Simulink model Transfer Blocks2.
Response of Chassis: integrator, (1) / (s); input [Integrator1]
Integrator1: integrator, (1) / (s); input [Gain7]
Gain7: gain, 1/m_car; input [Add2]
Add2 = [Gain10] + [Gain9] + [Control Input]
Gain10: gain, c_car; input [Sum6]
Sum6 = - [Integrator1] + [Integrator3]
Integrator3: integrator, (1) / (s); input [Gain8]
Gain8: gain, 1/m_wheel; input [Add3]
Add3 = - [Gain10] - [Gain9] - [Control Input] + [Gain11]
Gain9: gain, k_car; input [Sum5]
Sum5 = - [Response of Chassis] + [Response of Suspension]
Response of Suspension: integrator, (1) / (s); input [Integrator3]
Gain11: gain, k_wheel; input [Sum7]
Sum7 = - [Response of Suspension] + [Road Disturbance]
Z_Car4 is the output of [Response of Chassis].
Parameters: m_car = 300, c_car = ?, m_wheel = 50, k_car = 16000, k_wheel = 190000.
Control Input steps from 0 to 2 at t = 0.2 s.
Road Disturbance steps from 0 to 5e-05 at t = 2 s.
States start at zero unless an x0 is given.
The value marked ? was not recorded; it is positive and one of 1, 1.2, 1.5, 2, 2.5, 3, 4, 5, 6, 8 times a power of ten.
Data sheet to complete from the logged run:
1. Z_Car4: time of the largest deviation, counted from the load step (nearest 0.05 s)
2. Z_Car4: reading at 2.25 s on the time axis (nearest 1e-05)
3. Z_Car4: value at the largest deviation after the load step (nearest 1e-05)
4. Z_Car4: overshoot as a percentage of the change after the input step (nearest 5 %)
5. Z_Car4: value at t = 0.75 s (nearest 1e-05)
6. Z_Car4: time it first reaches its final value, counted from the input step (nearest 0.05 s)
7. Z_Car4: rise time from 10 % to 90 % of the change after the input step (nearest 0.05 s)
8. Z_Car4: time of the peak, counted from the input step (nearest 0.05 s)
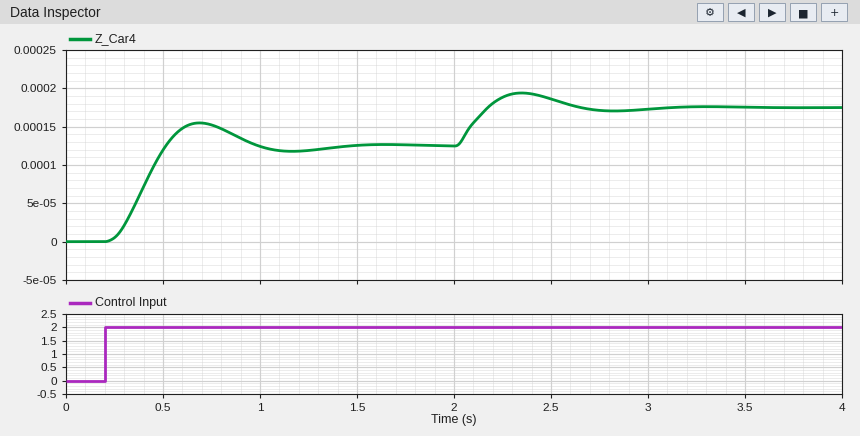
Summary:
0.35 s
0.00019
0.00019
25 %
0.00015
0.30 s
0.20 s
0.50 s
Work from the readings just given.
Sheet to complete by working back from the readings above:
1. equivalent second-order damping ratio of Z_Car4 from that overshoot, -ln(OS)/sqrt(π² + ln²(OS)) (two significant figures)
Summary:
0.40
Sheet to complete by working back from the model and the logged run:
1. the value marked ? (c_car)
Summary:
2000
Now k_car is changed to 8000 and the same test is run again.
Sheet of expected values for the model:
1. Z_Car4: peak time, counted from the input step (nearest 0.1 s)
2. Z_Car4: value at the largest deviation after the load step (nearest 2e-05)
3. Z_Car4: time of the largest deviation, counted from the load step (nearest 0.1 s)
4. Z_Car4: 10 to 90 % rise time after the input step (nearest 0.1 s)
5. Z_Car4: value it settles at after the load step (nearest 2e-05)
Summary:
0.8 s
0.00032
0.4 s
0.4 s
0.00030
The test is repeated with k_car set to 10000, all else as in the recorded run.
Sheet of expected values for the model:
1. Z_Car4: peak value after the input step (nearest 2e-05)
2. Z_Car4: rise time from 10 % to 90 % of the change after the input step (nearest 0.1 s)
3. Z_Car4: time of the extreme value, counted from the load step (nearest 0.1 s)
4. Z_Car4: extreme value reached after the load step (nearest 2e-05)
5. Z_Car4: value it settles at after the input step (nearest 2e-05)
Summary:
0.00022
0.3 s
0.4 s
0.00026
0.00020
